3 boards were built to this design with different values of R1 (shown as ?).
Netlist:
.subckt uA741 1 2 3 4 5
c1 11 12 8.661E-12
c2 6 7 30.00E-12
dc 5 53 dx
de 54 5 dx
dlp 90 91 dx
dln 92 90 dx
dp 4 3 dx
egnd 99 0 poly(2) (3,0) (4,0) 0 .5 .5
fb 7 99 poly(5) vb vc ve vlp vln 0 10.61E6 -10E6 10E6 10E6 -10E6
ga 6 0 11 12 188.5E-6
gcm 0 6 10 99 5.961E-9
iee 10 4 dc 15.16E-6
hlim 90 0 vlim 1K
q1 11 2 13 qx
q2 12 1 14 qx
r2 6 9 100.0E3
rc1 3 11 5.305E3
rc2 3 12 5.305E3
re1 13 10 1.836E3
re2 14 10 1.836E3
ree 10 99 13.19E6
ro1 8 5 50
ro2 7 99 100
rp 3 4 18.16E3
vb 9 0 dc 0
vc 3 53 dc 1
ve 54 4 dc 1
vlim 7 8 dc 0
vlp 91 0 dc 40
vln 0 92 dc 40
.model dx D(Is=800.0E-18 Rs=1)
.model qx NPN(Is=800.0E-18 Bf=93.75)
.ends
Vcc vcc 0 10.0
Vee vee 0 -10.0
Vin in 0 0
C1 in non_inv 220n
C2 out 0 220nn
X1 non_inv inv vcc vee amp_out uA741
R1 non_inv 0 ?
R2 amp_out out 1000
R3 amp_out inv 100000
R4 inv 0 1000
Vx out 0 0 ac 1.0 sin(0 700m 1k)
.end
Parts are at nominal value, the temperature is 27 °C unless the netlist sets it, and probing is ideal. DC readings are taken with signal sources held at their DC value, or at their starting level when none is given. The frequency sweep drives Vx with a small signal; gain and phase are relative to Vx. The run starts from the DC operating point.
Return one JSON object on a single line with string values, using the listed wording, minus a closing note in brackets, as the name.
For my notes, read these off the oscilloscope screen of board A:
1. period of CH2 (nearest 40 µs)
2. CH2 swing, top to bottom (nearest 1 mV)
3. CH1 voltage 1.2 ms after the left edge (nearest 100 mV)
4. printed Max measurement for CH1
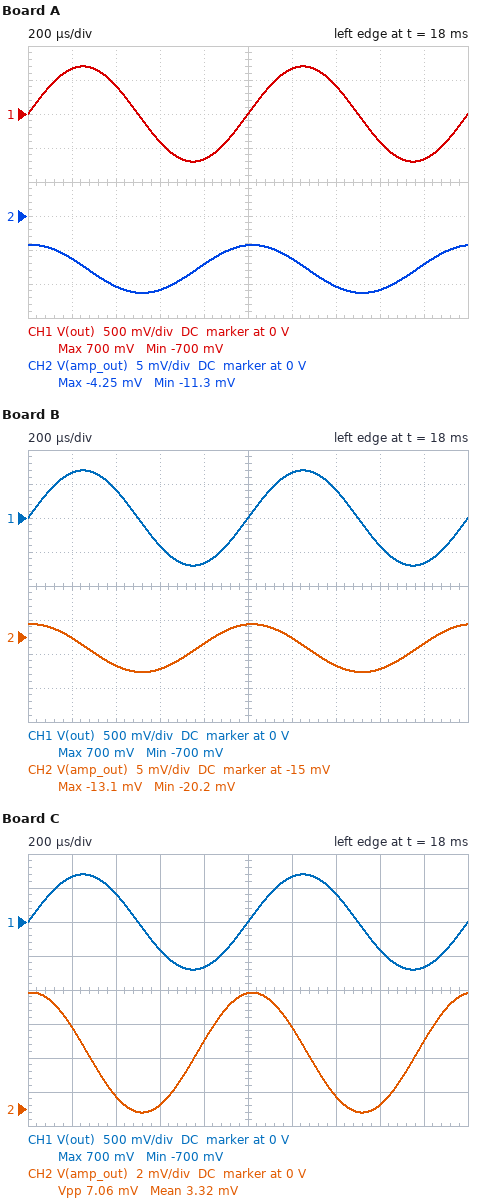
{"period of CH2": "1.00 ms", "CH2 swing, top to bottom": "7 mV", "CH1 voltage 1.2 ms after the left edge": "700 mV", "printed Max measurement for CH1": "700 mV"}
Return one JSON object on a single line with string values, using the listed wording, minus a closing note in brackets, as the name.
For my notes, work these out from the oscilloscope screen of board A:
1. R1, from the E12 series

{"R1, from the E12 series": "2.2 kΩ"}
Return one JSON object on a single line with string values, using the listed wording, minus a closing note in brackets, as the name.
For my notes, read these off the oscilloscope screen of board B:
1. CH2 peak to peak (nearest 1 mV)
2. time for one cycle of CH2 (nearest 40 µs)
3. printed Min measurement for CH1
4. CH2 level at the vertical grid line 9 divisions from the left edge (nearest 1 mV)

{"CH2 peak to peak": "7 mV", "time for one cycle of CH2": "1.00 ms", "printed Min measurement for CH1": "-700 mV", "CH2 level at the vertical grid line 9 divisions from the left edge": "-16 mV"}
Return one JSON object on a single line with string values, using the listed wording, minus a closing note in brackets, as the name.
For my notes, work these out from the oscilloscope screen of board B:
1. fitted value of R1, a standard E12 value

{"fitted value of R1, a standard E12 value": "3.3 kΩ"}
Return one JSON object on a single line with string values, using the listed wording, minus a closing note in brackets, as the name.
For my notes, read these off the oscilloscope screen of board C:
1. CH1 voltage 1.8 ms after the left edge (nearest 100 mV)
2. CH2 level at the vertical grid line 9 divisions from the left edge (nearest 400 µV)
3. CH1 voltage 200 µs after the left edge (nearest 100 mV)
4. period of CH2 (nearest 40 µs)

{"CH1 voltage 1.8 ms after the left edge": "-700 mV", "CH2 level at the vertical grid line 9 divisions from the left edge": "4.0 mV", "CH1 voltage 200 µs after the left edge": "700 mV", "period of CH2": "1.00 ms"}
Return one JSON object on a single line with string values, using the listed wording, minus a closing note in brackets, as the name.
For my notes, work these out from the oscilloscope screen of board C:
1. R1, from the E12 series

{"R1, from the E12 series": "820 Ω"}
